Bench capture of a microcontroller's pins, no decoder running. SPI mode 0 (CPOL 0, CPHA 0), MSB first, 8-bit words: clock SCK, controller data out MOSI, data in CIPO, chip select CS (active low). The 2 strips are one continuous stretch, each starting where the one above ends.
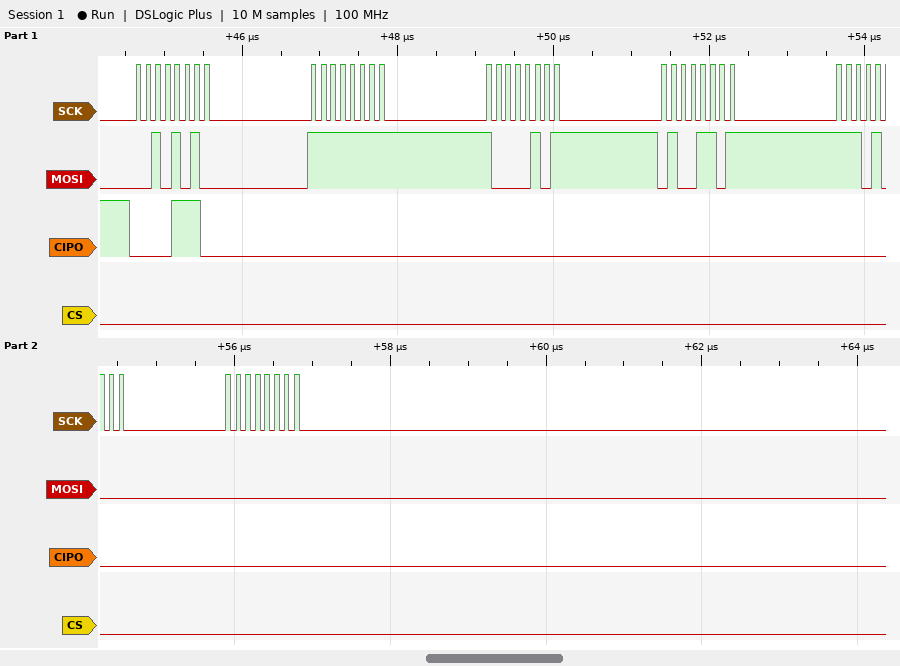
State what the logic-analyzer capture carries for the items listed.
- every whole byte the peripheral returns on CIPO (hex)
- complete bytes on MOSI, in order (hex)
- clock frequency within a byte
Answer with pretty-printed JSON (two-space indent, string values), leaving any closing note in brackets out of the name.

{
  "every whole byte the peripheral returns on CIPO": "0E 00 00 00 00 00",
  "complete bytes on MOSI, in order": "2A FF 85 4D E8 00",
  "clock frequency within a byte": "8 MHz"
}
